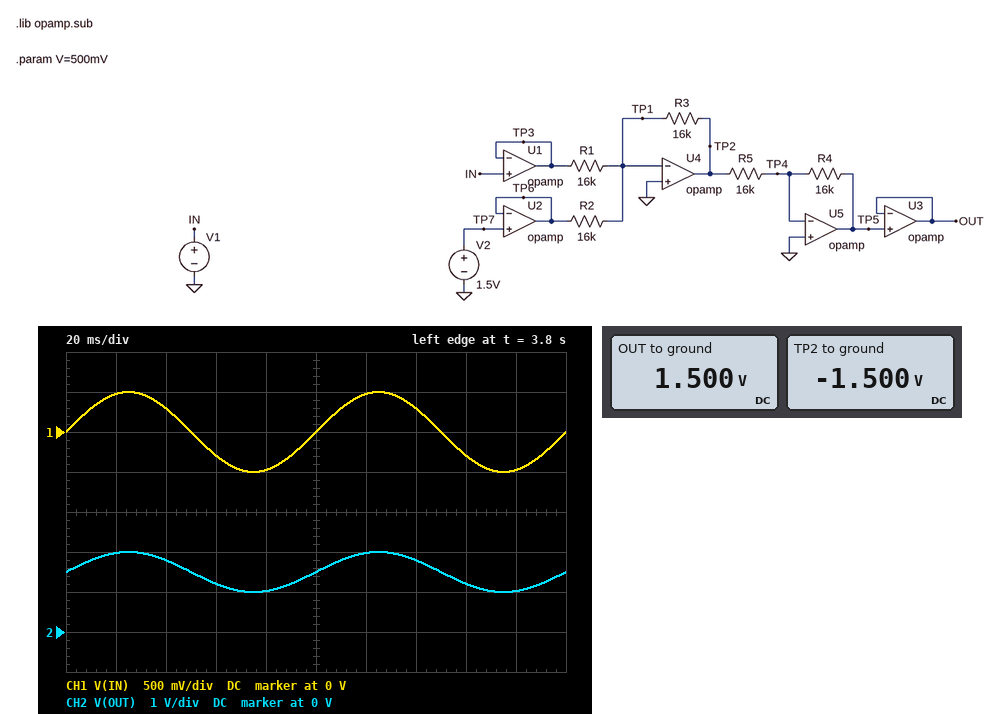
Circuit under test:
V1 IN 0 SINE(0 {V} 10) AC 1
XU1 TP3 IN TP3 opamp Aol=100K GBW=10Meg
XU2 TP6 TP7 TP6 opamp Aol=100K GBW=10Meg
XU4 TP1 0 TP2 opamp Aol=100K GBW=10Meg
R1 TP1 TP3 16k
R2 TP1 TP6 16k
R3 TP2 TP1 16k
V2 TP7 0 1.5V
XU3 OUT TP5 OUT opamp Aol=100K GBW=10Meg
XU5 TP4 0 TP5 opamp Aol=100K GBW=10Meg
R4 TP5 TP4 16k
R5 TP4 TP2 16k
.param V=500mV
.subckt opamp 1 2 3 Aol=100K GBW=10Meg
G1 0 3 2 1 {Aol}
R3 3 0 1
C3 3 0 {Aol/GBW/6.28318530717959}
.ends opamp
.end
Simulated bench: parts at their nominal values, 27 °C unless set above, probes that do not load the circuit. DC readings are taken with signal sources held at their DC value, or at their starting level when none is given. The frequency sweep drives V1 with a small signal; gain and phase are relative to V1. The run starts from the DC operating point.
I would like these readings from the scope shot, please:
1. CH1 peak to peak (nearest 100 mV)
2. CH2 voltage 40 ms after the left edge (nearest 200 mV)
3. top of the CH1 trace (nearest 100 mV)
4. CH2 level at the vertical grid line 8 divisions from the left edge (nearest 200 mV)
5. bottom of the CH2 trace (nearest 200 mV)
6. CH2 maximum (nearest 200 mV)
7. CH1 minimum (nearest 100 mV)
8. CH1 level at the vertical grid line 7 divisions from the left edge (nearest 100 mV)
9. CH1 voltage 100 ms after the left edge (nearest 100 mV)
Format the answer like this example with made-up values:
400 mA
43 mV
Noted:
1.0 V
1.8 V
500 mV
1.2 V
1.0 V
2.0 V
-500 mV
300 mV
0 V
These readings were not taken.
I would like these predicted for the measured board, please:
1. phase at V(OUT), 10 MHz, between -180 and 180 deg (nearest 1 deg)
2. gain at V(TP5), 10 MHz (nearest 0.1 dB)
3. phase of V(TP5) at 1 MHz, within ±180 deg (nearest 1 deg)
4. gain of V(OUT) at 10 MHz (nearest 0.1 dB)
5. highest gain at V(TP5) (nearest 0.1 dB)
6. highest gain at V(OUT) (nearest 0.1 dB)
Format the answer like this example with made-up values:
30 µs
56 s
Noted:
135 deg
-20.0 dB
-34 deg
-23.0 dB
0 dB
0 dB
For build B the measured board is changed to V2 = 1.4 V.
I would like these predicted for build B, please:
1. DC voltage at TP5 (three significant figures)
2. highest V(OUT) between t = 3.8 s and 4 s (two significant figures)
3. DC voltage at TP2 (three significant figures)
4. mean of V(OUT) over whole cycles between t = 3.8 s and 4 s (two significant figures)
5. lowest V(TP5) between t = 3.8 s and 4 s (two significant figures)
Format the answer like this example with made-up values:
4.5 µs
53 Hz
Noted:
1.40 V
1.9 V
-1.40 V
1.4 V
900 mV
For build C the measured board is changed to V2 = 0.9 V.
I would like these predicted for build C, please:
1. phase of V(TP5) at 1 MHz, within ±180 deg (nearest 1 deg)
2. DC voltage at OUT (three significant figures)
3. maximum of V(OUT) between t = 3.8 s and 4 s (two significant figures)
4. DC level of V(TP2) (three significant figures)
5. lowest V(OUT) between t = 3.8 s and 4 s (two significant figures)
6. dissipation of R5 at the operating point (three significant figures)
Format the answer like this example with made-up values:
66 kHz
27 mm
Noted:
-34 deg
900 mV
1.4 V
-900 mV
400 mV
50.6 µW
